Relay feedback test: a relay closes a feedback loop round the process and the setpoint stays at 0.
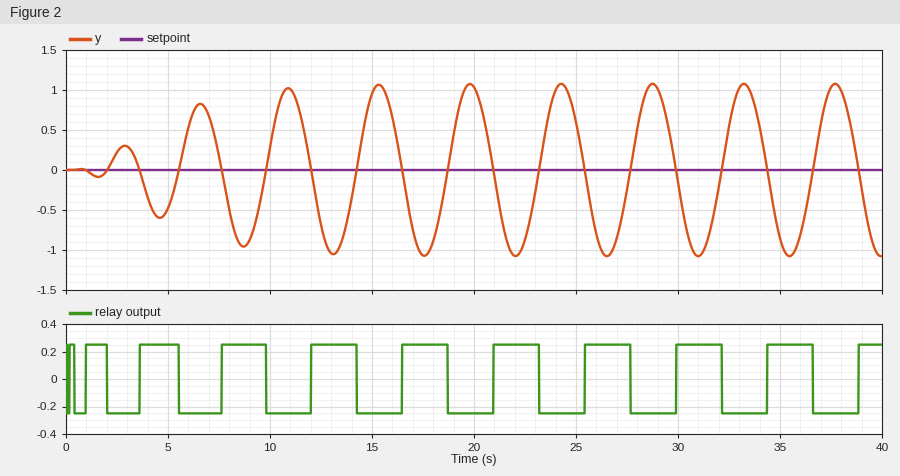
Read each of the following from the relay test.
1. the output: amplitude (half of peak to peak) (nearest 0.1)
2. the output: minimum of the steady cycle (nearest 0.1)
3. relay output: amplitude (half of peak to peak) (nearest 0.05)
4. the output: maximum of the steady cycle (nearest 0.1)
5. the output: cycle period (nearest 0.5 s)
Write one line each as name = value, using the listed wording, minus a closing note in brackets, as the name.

the output: amplitude (half of peak to peak) = 1.1
the output: minimum of the steady cycle = -1.1
relay output: amplitude (half of peak to peak) = 0.25
the output: maximum of the steady cycle = 1.1
the output: cycle period = 4.5 s
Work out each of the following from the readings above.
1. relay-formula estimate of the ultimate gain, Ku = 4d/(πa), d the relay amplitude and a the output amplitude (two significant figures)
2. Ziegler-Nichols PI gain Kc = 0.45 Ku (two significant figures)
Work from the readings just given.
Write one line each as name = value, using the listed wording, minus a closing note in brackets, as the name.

relay-formula estimate of the ultimate gain, Ku = 4d/(πa), d the relay amplitude and a the output amplitude = 0.29
Ziegler-Nichols PI gain Kc = 0.45 Ku = 0.13
